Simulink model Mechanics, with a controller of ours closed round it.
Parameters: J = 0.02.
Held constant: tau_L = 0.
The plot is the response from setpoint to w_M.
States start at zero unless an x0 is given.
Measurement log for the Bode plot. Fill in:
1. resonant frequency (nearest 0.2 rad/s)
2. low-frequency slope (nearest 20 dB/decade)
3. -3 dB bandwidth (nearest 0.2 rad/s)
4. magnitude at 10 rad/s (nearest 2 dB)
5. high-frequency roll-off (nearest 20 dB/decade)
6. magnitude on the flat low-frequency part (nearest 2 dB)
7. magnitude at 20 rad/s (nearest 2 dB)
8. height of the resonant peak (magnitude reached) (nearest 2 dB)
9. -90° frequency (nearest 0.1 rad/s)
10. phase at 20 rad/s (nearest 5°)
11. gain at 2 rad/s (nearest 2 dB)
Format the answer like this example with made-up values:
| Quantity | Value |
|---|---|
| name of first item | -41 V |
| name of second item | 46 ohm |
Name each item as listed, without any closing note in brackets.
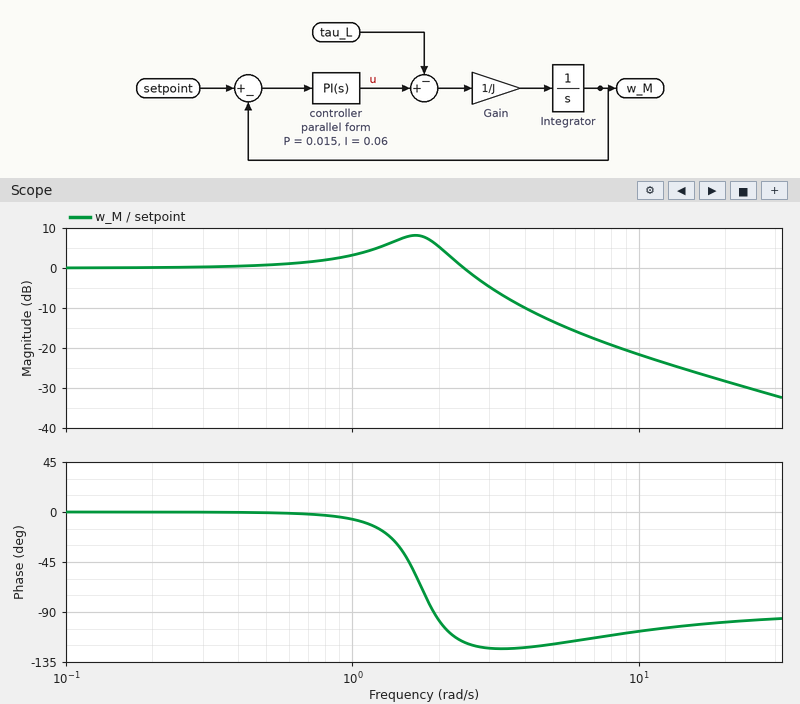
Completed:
| Quantity | Value |
|---|---|
| resonant frequency | 1.6 rad/s |
| low-frequency slope | 0 dB/decade |
| -3 dB bandwidth | 2.8 rad/s |
| magnitude at 10 rad/s | -22 dB |
| high-frequency roll-off | -20 dB/decade |
| magnitude on the flat low-frequency part | 0 dB |
| magnitude at 20 rad/s | -28 dB |
| height of the resonant peak (magnitude reached) | 8 dB |
| -90° frequency | 1.9 rad/s |
| phase at 20 rad/s | -100° |
| gain at 2 rad/s | 6 dB |
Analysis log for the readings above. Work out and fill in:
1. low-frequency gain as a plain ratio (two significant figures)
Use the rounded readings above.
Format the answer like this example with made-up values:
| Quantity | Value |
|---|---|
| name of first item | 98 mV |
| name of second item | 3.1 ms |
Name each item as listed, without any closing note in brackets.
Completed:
| Quantity | Value |
|---|---|
| low-frequency gain as a plain ratio | 1.0 |
